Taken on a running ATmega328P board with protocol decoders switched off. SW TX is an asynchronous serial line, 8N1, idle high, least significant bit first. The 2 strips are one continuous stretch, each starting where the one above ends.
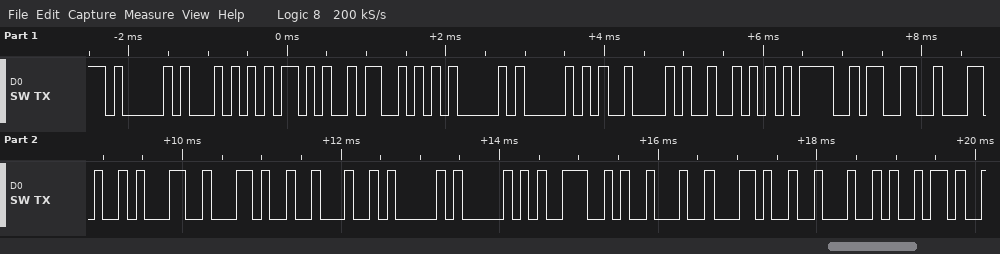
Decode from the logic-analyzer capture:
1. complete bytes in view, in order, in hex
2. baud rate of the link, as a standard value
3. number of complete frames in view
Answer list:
41 54 2B 53 41 50 42 52 3D 33 2C 31 2C 22 41 50 4E 22 2C 22 69
9600 baud
21
